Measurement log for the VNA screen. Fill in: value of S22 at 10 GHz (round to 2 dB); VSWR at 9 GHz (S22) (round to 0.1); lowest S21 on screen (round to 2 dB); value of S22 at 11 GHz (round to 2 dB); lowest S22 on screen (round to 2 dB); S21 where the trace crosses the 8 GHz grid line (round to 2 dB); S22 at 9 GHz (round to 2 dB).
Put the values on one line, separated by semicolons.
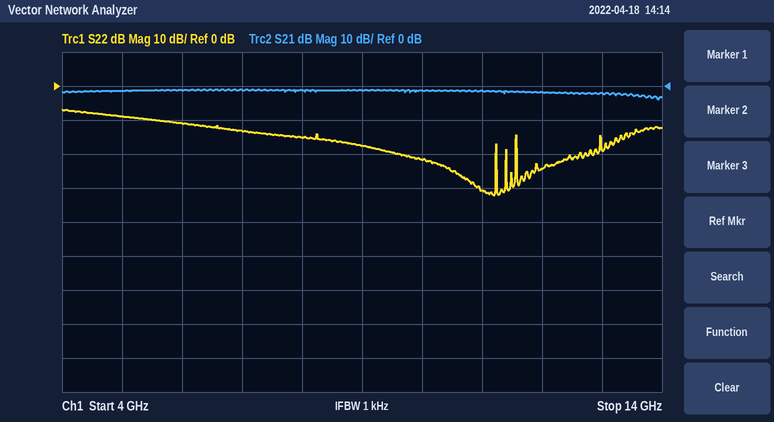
-22 dB; 1.3; -4 dB; -30 dB; -32 dB; -2 dB; -18 dB
